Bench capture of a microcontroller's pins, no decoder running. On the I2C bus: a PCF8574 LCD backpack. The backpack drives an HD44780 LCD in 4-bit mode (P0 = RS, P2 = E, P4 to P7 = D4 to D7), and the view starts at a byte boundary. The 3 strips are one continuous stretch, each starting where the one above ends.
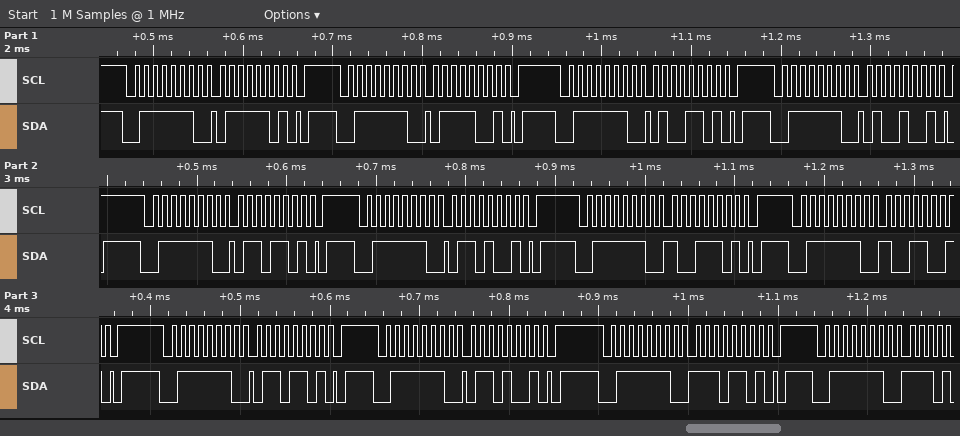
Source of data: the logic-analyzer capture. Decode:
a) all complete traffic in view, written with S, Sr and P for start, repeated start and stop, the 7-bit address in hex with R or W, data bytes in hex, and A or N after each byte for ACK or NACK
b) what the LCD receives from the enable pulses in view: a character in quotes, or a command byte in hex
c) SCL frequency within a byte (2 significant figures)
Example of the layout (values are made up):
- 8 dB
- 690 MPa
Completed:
- S 3FW A 7D A P S 3FW A 79 A P S 3FW A 4D A P S 3FW A 49 A P S 3FW A 6D A P S 3FW A 69 A P S 3FW A 9D A P S 3FW A 99 A P S 3FW A 6D A P S 3FW A 69 A P S 3FW A ED A P S 3FW A
- 't' 'i'
- 100 kHz
